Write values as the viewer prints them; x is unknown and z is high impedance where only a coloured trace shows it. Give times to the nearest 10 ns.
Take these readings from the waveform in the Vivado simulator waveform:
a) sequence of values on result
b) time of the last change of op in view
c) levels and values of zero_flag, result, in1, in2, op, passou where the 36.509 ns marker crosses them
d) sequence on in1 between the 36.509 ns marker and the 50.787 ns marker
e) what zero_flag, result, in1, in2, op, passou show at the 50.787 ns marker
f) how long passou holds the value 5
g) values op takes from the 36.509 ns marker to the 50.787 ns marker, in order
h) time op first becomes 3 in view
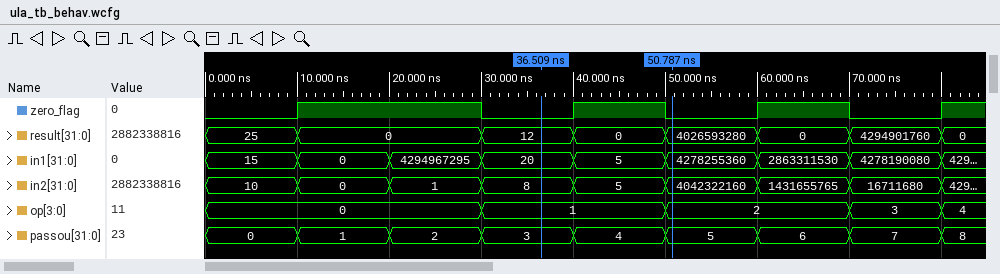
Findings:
25, 0, 12, 0, 4026593280, 0, 4294901760, 0
80 ns
zero_flag=0, result=12, in1=20, in2=8, op=1, passou=3
20, 5, 4278255360
zero_flag=0, result=4026593280, in1=4278255360, in2=4042322160, op=2, passou=5
10 ns
1, 2
70 ns
